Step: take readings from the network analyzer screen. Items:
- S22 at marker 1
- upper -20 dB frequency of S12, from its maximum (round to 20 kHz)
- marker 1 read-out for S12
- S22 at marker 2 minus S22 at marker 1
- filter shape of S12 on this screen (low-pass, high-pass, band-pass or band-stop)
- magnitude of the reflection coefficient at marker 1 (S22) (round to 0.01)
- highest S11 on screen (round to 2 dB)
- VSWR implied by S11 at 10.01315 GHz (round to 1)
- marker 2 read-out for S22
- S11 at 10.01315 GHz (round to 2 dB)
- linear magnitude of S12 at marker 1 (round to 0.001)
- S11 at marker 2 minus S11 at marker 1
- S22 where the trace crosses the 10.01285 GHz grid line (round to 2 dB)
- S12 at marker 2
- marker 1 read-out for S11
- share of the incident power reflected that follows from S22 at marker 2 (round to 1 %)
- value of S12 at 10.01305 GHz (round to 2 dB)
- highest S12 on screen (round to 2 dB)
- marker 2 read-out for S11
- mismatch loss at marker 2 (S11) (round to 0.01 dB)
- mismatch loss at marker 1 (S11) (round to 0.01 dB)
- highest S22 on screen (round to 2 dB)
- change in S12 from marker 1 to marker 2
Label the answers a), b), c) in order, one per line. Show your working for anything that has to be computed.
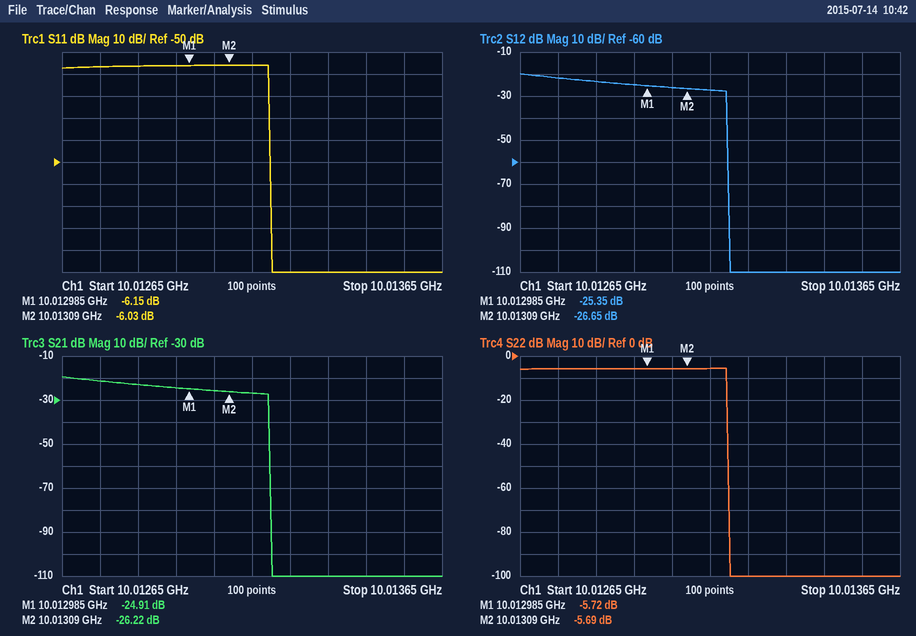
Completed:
a) -5.72 dB
b) 10.01320 GHz
c) -25.35 dB
d) -5.69 − (-5.72) = 0.03 dB
e) low-pass
f) 10^(-5.72/20) ≈ 0.52
g) -6 dB
h) |Γ| = 10^(-6/20) = 0.5012; VSWR = (1 + 0.5012)/(1 − 0.5012) ≈ 3
i) -5.69 dB
j) -6 dB
k) 10^(-25.35/20) ≈ 0.054
l) -6.03 − (-6.15) = 0.12 dB
m) -6 dB
n) -26.65 dB
o) -6.15 dB
p) 10^(-5.69/10) ≈ 27 %
q) -26 dB
r) -20 dB
s) -6.03 dB
t) −10 log10(1 − 10^(-6.03/10)) ≈ 1.25 dB
u) −10 log10(1 − 10^(-6.15/10)) ≈ 1.21 dB
v) -6 dB
w) -26.65 − (-25.35) = -1.30 dB
